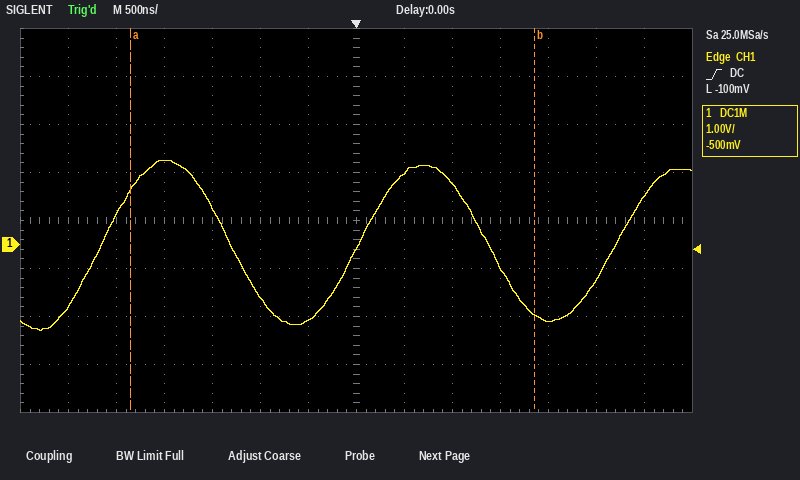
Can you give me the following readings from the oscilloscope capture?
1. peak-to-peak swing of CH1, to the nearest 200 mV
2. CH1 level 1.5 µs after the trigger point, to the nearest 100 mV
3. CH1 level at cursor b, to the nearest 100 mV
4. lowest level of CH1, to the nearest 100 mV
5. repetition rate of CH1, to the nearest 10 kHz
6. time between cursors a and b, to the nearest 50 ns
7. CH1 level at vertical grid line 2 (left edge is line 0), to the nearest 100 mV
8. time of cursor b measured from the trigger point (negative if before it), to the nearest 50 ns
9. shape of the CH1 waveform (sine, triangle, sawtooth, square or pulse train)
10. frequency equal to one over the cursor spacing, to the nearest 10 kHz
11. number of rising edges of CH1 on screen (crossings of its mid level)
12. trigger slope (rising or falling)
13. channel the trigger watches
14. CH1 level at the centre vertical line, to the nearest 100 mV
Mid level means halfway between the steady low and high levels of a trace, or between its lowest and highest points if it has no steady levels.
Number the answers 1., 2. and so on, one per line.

1. 3.6 V
2. -500 mV
3. -1.5 V
4. -1.8 V
5. 370 kHz
6. 4.20 µs
7. 600 mV
8. +1.85 µs
9. sine
10. 240 kHz
11. 3
12. rising
13. CH1
14. -100 mV
